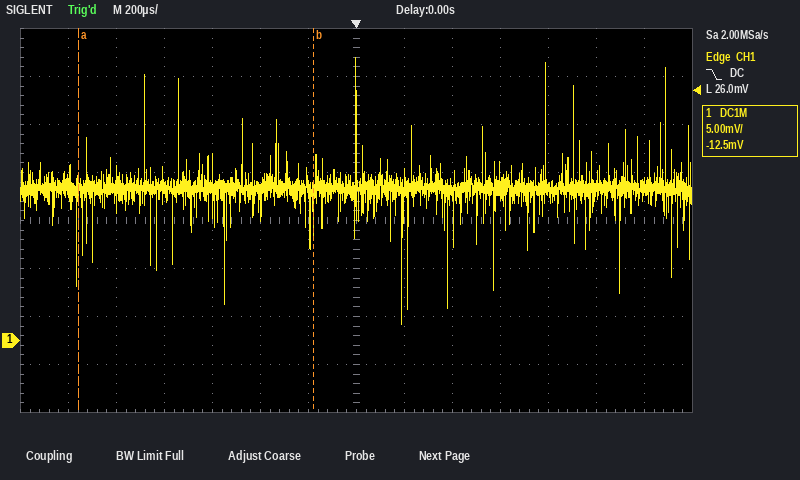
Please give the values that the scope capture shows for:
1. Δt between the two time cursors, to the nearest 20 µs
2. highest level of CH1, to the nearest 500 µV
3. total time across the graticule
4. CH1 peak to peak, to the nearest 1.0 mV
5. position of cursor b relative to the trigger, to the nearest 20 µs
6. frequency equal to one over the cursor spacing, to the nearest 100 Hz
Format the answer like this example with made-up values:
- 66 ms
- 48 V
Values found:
- 980 µs
- 29.5 mV
- 2.8 ms
- 28.0 mV
- -180 µs
- 1.0 kHz
